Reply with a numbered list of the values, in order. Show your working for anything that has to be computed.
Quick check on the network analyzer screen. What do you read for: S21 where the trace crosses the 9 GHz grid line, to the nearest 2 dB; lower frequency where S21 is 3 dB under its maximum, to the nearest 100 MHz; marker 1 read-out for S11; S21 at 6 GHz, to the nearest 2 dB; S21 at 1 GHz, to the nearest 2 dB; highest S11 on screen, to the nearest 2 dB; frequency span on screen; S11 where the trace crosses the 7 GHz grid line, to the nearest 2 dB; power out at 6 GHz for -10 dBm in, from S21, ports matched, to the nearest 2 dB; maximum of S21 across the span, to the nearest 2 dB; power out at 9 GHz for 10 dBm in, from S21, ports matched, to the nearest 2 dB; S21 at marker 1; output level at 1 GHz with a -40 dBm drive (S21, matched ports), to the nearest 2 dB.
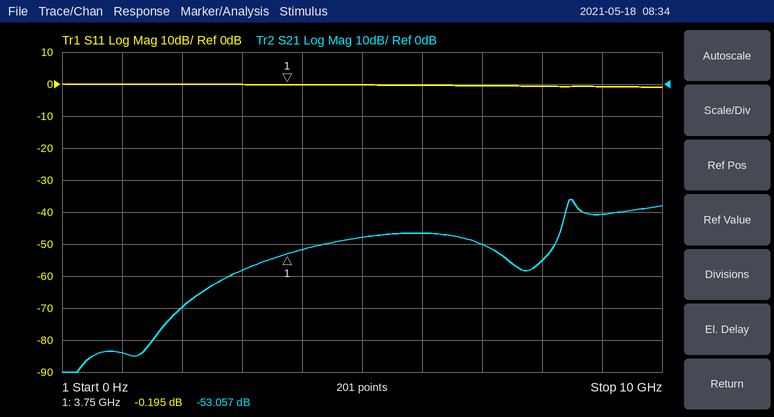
1. -40 dB
2. 8.4 GHz
3. -0.195 dB
4. -46 dB
5. -84 dB
6. 0 dB
7. 10 GHz
8. 0 dB
9. -10 dBm + (-46 dB) = -56 dBm
10. -36 dB
11. 10 dBm + (-40 dB) = -30 dBm
12. -53.057 dB
13. -40 dBm + (-84 dB) = -124 dBm
